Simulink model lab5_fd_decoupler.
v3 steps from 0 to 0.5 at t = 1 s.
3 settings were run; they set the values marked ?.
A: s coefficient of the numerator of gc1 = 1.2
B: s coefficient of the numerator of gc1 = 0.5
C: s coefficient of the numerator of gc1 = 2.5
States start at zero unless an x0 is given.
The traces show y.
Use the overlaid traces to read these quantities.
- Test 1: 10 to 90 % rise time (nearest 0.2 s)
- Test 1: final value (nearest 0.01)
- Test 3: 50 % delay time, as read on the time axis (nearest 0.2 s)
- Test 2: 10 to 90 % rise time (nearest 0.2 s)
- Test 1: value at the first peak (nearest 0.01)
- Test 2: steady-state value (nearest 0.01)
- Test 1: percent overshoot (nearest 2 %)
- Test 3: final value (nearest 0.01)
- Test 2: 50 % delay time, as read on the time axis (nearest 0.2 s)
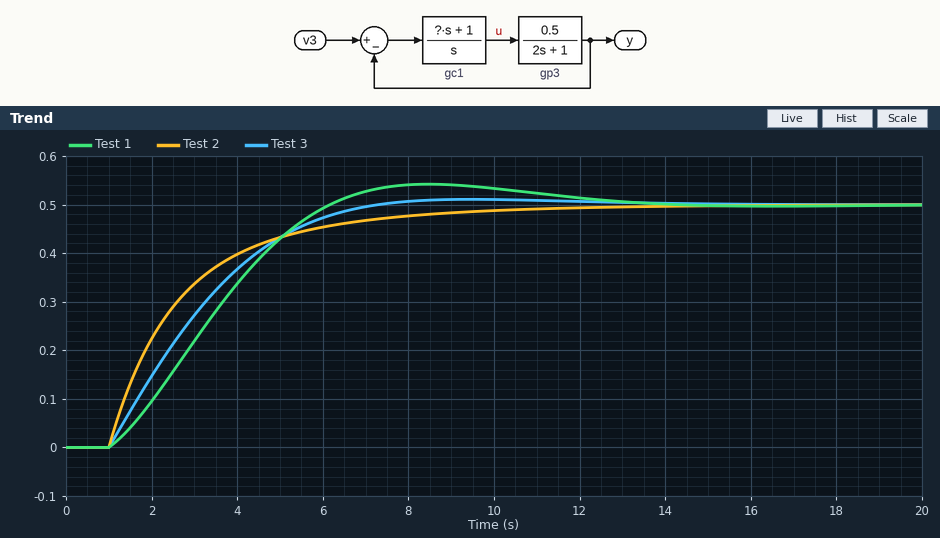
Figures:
3.6 s
0.50
2.8 s
4.6 s
0.54
0.50
8 %
0.50
2.2 s
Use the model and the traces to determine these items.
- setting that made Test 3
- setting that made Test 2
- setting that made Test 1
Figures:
A
C
B
